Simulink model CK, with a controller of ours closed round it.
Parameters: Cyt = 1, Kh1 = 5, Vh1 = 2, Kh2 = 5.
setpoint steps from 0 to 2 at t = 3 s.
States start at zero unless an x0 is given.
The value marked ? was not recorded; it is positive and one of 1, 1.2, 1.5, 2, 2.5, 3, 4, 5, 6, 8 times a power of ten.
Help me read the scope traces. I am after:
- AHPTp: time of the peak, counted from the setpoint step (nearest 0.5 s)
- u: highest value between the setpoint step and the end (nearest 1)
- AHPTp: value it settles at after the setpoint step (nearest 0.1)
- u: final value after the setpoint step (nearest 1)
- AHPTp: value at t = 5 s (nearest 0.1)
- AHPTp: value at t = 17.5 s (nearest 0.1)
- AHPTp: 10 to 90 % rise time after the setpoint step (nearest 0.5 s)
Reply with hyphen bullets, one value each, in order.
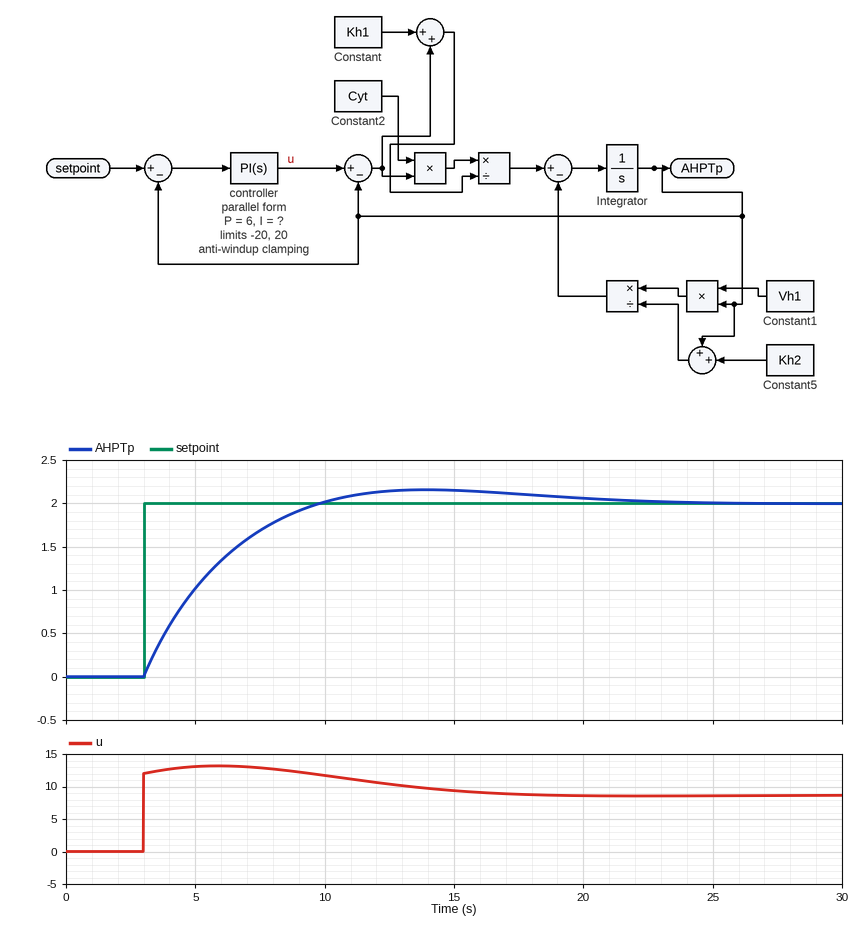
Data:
- 11.0 s
- 13
- 2.0
- 9
- 1.0
- 2.1
- 5.0 s
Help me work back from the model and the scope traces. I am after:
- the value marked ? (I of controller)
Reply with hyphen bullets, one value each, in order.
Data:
- 2.5
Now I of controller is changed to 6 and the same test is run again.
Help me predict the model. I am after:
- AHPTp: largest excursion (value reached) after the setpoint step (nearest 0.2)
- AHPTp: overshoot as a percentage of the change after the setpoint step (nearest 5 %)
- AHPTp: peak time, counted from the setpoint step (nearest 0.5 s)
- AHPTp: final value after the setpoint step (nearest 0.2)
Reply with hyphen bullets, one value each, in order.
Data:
- 2.4
- 20 %
- 8.5 s
- 2.0
